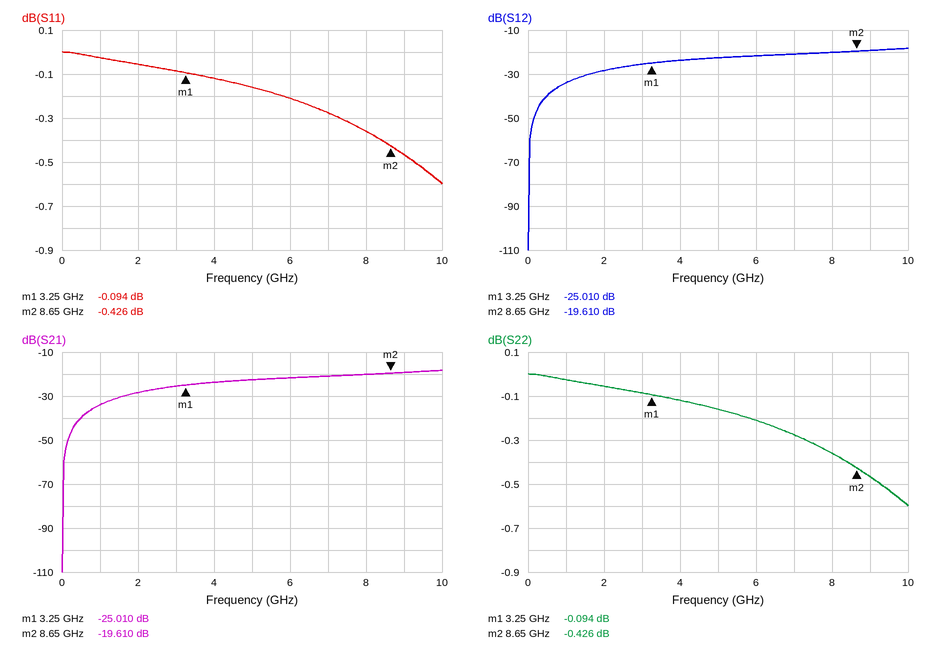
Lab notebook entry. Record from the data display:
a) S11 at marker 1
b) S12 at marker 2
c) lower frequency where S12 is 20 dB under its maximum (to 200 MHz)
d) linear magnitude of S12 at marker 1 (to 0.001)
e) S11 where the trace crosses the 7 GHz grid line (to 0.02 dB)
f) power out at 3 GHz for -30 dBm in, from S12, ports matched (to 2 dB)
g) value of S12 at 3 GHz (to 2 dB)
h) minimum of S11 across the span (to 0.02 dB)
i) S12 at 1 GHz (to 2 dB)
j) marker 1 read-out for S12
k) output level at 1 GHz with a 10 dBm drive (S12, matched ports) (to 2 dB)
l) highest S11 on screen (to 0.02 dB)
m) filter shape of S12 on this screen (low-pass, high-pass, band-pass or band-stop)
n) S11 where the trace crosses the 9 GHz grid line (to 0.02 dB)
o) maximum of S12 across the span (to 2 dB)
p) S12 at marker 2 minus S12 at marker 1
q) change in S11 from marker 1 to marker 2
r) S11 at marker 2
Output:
-0.094 dB
-19.610 dB
600 MHz
0.056
-0.28 dB
-56 dBm
-26 dB
-0.60 dB
-34 dB
-25.010 dB
-24 dBm
0.00 dB
high-pass
-0.46 dB
-18 dB
5.400 dB
-0.332 dB
-0.426 dB
